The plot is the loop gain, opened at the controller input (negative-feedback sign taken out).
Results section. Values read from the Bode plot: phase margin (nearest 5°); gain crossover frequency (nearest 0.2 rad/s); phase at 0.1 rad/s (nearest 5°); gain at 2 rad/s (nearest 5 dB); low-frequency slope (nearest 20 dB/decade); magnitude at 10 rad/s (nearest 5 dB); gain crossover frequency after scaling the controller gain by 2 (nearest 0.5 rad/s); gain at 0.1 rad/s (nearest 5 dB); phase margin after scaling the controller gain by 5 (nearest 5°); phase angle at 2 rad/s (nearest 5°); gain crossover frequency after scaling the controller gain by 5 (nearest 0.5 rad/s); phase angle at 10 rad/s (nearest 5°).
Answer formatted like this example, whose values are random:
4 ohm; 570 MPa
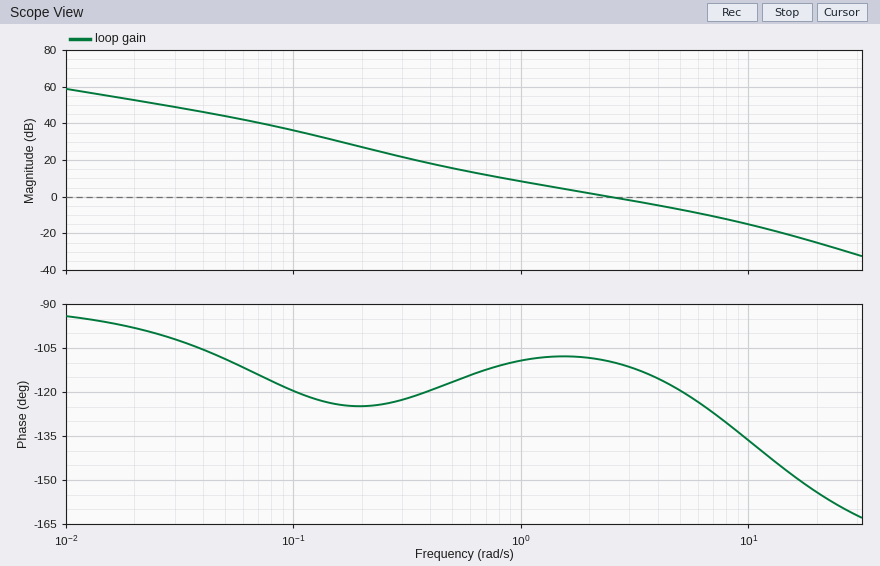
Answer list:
70°; 2.4 rad/s; -120°; 0 dB; -20 dB/decade; -15 dB; 4.5 rad/s; 35 dB; 45°; -110°; 9.0 rad/s; -135°
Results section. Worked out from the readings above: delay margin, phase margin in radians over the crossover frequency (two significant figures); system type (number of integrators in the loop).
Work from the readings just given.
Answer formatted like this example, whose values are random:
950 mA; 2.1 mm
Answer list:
0.51 s; 1
